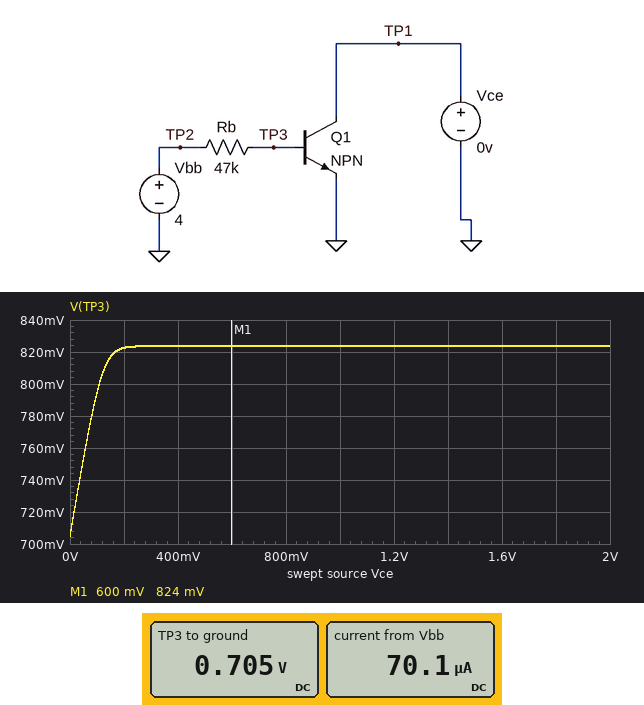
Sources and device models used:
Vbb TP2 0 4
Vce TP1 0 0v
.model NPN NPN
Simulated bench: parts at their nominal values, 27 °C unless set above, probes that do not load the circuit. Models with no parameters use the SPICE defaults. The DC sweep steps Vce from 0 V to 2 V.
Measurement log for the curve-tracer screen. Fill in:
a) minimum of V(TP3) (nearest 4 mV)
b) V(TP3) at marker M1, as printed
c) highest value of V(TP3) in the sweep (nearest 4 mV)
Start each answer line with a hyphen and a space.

- 704 mV
- 824 mV
- 824 mV
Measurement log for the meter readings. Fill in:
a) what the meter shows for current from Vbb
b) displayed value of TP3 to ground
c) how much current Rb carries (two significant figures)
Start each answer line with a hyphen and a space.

- 70.1 µA
- 0.705 V
- 70 µA
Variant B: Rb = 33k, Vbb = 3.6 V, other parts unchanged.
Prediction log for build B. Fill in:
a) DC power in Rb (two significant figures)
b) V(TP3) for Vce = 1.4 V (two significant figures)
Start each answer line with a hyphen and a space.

- 250 µW
- 830 mV
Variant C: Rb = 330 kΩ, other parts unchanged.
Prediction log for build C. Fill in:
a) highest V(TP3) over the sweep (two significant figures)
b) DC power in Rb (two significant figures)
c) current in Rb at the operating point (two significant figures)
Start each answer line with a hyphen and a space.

- 770 mV
- 34 µW
- 10 µA
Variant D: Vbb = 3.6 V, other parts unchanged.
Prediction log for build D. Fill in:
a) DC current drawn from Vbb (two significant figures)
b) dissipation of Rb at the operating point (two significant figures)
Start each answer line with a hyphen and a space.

- 62 µA
- 180 µW
